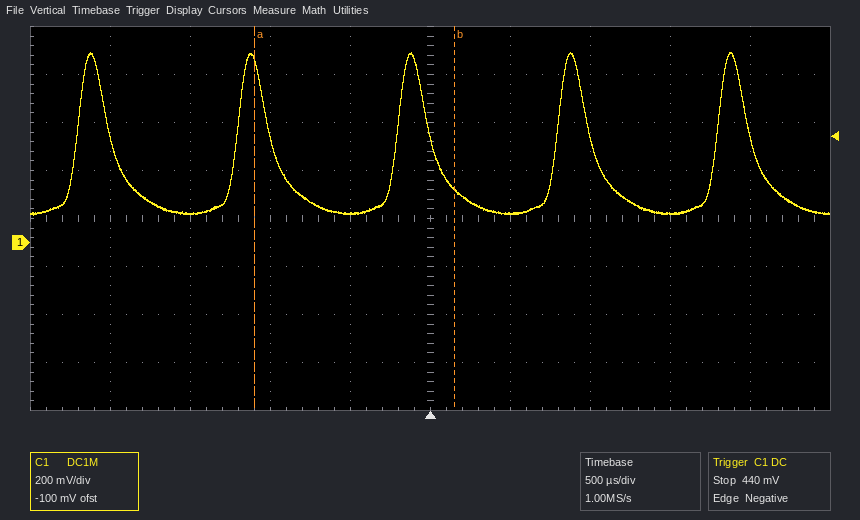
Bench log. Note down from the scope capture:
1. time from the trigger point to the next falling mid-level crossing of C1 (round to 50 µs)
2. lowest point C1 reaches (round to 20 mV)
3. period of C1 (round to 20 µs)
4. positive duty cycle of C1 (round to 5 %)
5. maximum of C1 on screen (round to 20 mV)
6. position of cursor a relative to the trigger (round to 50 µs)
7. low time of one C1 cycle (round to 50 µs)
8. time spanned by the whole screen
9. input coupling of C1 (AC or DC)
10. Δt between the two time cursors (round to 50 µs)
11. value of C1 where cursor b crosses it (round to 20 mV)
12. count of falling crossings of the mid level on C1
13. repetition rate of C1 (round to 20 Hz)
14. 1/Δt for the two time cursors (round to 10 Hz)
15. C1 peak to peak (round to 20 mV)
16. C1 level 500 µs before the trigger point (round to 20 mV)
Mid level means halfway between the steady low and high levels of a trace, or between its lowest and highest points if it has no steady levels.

1.00 ms
120 mV
1.00 ms
20 %
800 mV
-1.10 ms
800 µs
5 ms
DC
1.25 ms
220 mV
5
1.00 kHz
800 Hz
680 mV
120 mV
